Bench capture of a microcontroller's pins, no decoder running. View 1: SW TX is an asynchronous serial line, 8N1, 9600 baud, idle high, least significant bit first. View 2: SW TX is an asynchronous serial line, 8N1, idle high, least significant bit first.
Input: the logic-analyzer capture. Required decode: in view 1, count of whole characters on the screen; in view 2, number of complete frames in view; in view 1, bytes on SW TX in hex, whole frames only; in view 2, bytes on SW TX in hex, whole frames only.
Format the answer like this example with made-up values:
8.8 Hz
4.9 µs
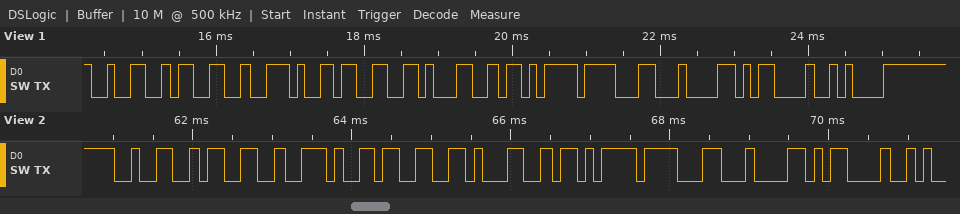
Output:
10
9
32 33 2E 33 31 EB 8F 84 0D 0A
0x32 0x33 0x2E 0x33 0x31 0xEB 0x8F 0x84 0x0D
